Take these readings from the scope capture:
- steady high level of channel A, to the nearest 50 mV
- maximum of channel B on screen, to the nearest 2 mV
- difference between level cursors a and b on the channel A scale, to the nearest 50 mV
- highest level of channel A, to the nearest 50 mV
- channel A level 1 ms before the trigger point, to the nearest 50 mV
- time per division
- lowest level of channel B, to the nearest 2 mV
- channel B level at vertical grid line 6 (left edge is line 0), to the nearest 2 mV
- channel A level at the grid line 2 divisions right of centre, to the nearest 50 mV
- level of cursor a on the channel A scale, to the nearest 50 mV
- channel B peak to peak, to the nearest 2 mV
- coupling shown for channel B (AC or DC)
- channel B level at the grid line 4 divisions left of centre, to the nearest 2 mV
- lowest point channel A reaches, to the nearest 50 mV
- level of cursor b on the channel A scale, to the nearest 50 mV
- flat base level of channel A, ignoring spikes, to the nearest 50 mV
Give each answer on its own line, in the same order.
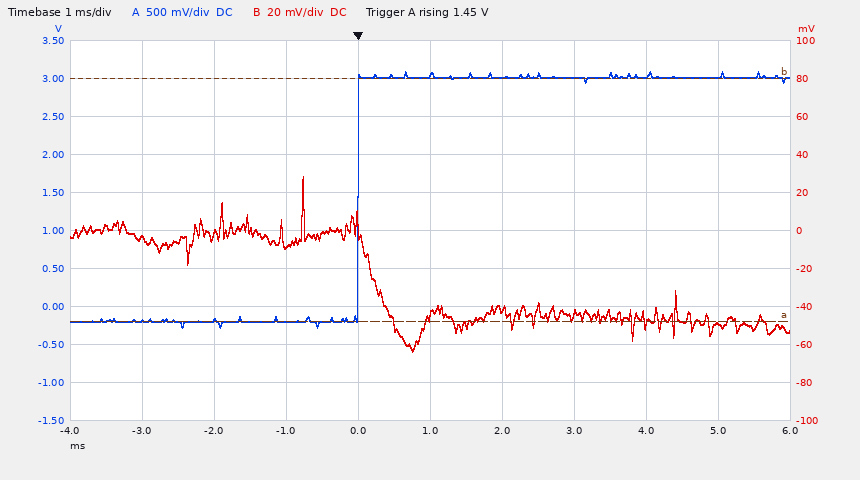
3.00 V
28 mV
3.20 V
3.10 V
-200 mV
1 ms
-64 mV
-42 mV
3.00 V
-200 mV
92 mV
DC
-4 mV
-300 mV
3.00 V
-200 mV
